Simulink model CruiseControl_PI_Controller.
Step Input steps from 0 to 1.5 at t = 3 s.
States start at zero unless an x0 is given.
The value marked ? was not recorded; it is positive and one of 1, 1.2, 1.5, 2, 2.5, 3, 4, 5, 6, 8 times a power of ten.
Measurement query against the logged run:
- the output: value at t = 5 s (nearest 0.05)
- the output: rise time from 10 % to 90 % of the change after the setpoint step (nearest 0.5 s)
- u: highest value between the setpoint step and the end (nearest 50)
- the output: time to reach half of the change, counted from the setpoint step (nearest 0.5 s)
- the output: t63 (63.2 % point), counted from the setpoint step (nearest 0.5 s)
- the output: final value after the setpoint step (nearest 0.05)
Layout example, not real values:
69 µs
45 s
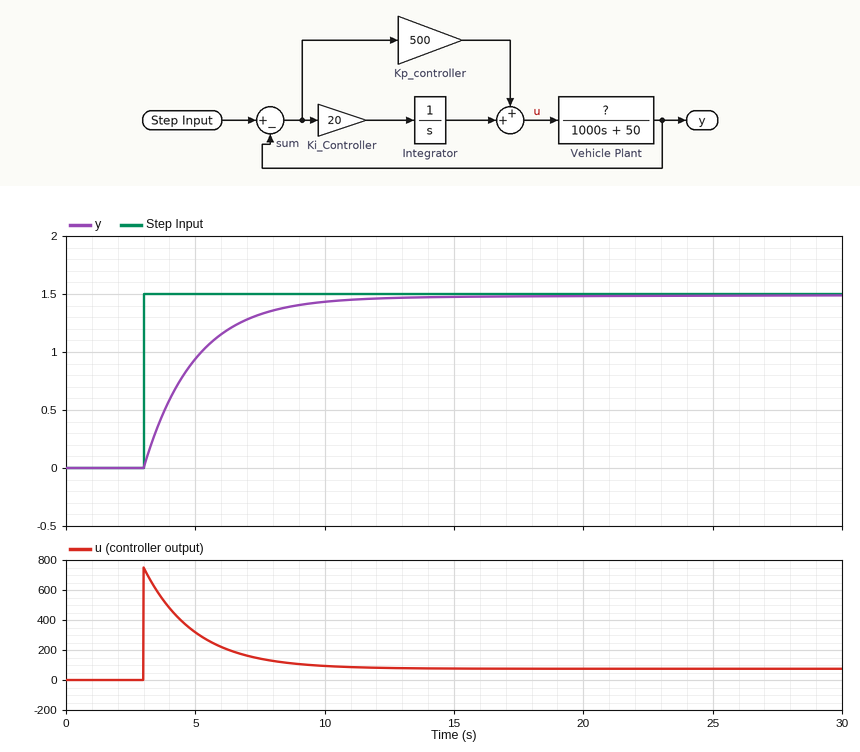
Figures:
0.95
4.5 s
750
1.5 s
2.0 s
1.50
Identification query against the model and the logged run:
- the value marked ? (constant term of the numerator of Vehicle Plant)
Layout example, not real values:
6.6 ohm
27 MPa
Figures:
1
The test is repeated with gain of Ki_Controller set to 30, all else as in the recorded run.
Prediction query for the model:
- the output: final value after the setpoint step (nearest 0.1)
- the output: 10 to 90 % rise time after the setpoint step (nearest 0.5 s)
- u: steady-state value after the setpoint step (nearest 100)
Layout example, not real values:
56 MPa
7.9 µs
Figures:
1.5
4.0 s
100
